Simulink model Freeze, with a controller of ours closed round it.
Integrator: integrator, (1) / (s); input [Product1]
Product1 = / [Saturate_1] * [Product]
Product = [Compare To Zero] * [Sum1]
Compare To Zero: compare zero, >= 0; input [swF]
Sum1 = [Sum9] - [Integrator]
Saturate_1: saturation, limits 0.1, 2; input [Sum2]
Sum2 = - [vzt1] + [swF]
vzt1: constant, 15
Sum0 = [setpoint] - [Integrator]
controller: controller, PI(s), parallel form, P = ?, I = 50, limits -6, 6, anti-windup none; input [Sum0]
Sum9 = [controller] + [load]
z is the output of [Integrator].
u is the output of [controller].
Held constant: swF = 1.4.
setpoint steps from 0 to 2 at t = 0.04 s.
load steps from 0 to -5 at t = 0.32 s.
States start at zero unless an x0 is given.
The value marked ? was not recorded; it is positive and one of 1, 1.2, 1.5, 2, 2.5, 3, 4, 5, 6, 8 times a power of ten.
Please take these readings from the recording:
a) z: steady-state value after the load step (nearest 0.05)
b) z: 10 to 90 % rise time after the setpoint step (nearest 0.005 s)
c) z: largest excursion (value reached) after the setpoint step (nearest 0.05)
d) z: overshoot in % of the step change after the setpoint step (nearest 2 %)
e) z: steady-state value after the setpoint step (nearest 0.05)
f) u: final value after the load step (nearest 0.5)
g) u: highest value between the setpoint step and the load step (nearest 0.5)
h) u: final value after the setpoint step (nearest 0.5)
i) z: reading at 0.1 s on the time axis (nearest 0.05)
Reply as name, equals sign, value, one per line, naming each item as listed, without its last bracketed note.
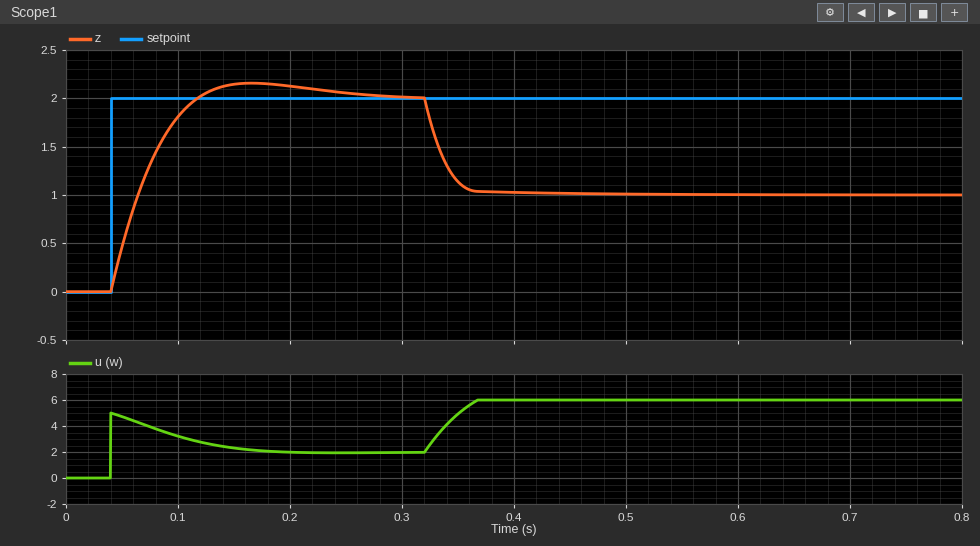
z: steady-state value after the load step = 1.00
z: 10 to 90 % rise time after the setpoint step = 0.055 s
z: largest excursion (value reached) after the setpoint step = 2.15
z: overshoot in % of the step change after the setpoint step = 8 %
z: steady-state value after the setpoint step = 2.00
u: final value after the load step = 6.0
u: highest value between the setpoint step and the load step = 5.0
u: final value after the setpoint step = 2.0
z: reading at 0.1 s on the time axis = 1.80
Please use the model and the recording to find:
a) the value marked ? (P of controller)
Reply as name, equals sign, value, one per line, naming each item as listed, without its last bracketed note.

the value marked ? = 2.5
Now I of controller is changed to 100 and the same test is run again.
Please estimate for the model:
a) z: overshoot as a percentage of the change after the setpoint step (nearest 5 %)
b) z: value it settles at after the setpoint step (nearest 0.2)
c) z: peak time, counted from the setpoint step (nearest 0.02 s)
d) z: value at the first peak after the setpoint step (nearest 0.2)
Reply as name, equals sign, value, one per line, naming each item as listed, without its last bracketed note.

z: overshoot as a percentage of the change after the setpoint step = 20 %
z: value it settles at after the setpoint step = 2.0
z: peak time, counted from the setpoint step = 0.08 s
z: value at the first peak after the setpoint step = 2.4
